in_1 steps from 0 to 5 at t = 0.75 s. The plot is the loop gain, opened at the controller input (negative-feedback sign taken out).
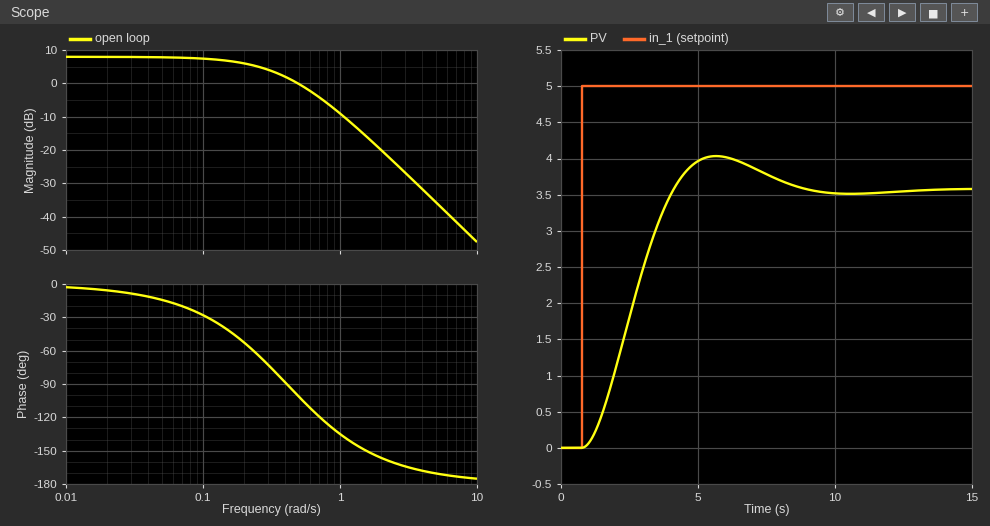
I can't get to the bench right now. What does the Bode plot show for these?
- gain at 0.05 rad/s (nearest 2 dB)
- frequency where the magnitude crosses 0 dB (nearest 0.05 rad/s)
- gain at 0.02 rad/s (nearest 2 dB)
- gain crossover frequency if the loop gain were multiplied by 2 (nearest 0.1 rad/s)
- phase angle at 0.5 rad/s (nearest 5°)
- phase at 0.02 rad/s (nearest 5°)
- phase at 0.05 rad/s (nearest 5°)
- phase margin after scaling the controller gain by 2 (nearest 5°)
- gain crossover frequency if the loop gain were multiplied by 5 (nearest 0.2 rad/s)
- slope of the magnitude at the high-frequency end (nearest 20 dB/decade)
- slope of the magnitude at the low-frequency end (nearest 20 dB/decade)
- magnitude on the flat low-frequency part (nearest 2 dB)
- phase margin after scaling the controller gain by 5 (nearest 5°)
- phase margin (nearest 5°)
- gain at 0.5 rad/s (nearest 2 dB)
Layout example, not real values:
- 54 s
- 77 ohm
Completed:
- 8 dB
- 0.50 rad/s
- 8 dB
- 0.8 rad/s
- -100°
- -5°
- -15°
- 55°
- 1.4 rad/s
- -40 dB/decade
- 0 dB/decade
- 8 dB
- 35°
- 80°
- 0 dB
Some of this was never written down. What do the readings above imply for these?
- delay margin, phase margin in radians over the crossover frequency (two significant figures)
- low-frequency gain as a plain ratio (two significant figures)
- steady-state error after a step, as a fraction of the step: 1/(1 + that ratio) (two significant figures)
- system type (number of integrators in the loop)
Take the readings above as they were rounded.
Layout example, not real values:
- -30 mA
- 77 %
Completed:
- 2.8 s
- 2.5
- 0.29
- 0
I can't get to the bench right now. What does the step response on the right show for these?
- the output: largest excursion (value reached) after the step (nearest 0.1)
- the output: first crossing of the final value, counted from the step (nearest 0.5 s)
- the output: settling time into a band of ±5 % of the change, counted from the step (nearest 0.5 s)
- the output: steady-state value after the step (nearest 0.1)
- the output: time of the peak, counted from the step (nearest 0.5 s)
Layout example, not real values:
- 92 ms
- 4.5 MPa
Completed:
- 4.0
- 3.5 s
- 7.0 s
- 3.6
- 5.0 s
